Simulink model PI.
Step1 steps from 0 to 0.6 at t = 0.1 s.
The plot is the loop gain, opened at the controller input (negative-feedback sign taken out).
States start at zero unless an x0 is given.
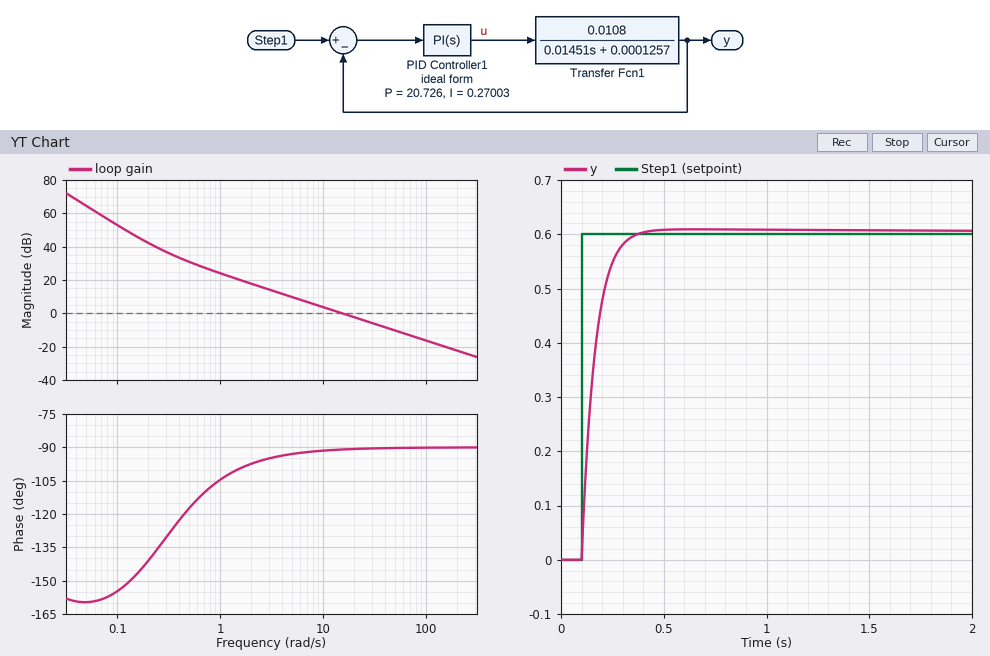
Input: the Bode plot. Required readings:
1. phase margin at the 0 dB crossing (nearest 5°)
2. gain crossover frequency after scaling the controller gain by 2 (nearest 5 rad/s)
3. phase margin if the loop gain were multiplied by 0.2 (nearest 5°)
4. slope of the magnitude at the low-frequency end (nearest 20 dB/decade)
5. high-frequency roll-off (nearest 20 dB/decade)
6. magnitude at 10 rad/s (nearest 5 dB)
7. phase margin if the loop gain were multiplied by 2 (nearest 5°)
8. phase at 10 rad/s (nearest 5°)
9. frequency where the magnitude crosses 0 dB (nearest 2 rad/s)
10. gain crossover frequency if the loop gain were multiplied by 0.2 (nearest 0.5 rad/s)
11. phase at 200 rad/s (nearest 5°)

90°
30 rad/s
85°
-40 dB/decade
-20 dB/decade
5 dB
90°
-90°
16 rad/s
3.0 rad/s
-90°
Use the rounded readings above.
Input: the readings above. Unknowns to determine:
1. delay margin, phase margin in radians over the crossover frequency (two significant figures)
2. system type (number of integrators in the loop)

0.098 s
2
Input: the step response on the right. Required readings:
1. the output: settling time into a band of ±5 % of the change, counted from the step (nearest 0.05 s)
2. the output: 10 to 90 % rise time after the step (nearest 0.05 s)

0.20 s
0.15 s
